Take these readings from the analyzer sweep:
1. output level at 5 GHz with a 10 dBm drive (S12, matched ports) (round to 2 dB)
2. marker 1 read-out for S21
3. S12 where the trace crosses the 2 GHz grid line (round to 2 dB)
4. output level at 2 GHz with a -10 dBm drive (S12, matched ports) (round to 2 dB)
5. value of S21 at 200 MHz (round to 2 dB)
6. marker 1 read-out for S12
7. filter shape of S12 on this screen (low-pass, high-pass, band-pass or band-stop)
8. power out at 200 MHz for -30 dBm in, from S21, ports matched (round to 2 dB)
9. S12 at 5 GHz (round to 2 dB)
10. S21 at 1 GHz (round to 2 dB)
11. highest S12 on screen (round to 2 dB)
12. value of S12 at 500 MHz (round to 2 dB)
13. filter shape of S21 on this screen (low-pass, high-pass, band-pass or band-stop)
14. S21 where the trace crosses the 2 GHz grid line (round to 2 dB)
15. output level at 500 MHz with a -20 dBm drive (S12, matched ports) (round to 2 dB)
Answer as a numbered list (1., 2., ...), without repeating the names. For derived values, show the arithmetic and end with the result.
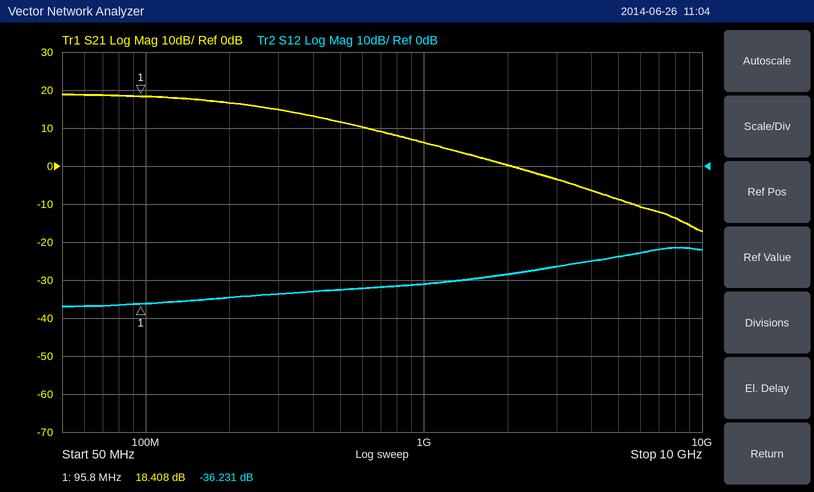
1. 10 dBm + (-24 dB) = -14 dBm
2. 18.408 dB
3. -28 dB
4. -10 dBm + (-28 dB) = -38 dBm
5. 16 dB
6. -36.231 dB
7. high-pass
8. -30 dBm + (16 dB) = -14 dBm
9. -24 dB
10. 6 dB
11. -22 dB
12. -32 dB
13. low-pass
14. 0 dB
15. -20 dBm + (-32 dB) = -52 dBm
